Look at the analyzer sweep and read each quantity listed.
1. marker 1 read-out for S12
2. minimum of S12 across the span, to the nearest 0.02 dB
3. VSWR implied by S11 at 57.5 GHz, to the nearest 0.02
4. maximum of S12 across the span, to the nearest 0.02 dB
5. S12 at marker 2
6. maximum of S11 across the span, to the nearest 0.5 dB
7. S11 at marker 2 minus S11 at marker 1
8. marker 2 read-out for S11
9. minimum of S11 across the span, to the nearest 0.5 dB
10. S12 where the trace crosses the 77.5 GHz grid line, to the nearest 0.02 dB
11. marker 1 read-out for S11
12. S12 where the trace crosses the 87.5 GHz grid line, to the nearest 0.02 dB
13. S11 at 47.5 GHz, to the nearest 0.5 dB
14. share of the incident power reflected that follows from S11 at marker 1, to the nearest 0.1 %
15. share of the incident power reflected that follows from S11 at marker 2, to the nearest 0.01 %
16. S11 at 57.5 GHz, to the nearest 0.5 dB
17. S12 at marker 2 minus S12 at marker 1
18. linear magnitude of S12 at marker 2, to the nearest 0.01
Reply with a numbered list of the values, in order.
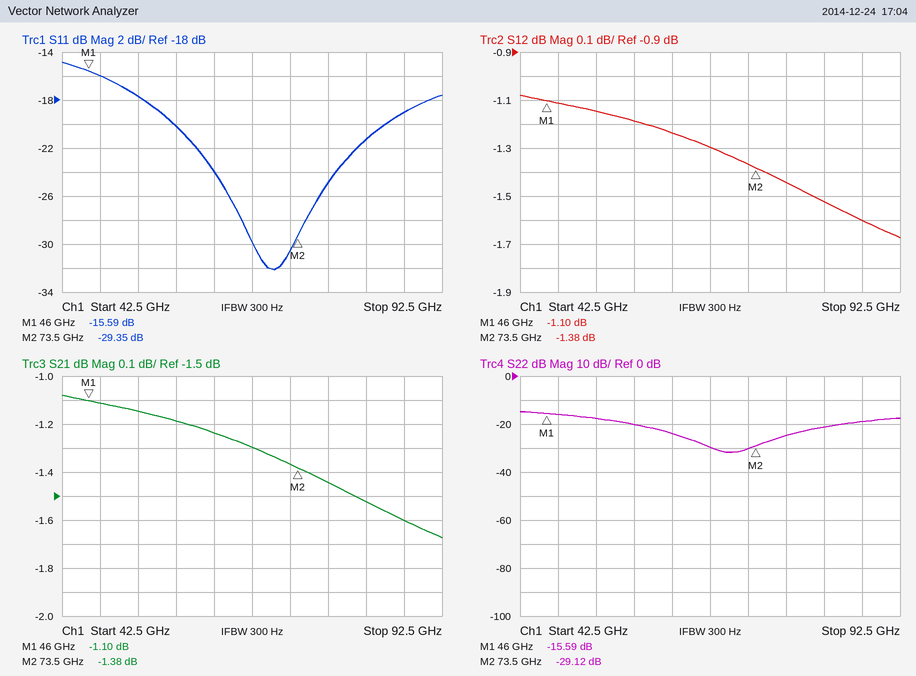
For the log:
1. -1.10 dB
2. -1.68 dB
3. 1.22
4. -1.08 dB
5. -1.38 dB
6. -15.0 dB
7. -13.76 dB
8. -29.35 dB
9. -32.0 dB
10. -1.44 dB
11. -15.59 dB
12. -1.60 dB
13. -16.0 dB
14. 2.8 %
15. 0.12 %
16. -20.0 dB
17. -0.28 dB
18. 0.85
